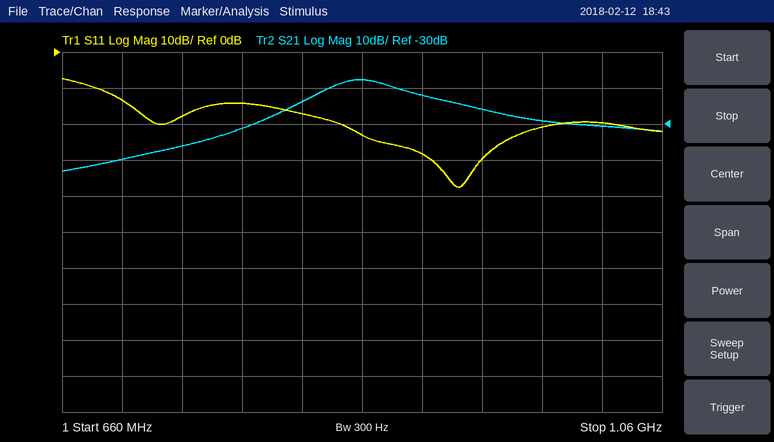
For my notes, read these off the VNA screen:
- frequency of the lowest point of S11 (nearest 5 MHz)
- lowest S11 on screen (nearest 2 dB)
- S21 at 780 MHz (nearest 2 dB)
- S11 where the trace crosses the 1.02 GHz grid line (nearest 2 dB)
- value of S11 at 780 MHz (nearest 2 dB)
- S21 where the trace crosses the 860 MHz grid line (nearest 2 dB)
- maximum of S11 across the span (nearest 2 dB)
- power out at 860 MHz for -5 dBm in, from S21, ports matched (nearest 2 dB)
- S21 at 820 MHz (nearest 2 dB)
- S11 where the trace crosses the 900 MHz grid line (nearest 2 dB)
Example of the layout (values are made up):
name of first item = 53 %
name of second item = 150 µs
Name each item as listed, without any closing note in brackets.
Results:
frequency of the lowest point of S11 = 925 MHz
lowest S11 on screen = -38 dB
S21 at 780 MHz = -32 dB
S11 where the trace crosses the 1.02 GHz grid line = -20 dB
value of S11 at 780 MHz = -14 dB
S21 where the trace crosses the 860 MHz grid line = -18 dB
maximum of S11 across the span = -8 dB
power out at 860 MHz for -5 dBm in, from S21, ports matched = -22 dBm
S21 at 820 MHz = -24 dB
S11 where the trace crosses the 900 MHz grid line = -28 dB
